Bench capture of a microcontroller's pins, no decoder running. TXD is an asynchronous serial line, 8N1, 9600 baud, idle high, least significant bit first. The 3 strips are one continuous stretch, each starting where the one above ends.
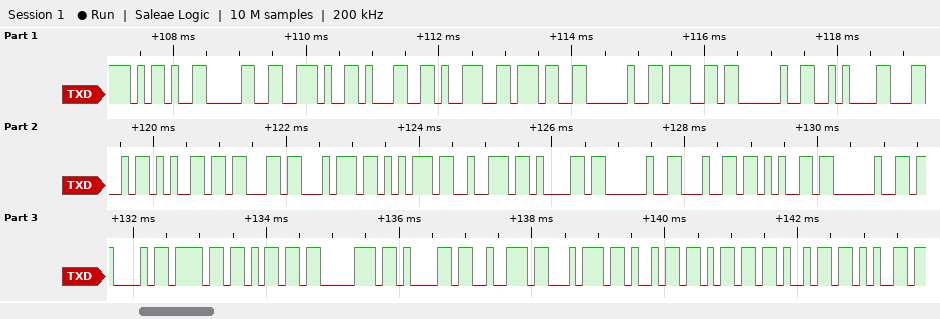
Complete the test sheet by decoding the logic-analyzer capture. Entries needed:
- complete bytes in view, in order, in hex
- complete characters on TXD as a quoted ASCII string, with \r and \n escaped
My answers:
0x2D 0x30 0x2E 0x31 0x39 0x37 0x20 0x67 0x20 0x0A 0x4C 0x65 0x63 0x74 0x75 0x72 0x61 0x20 0x64 0x65 0x20 0x43 0x6F 0x6D 0x70 0x61 0x72 0x74 0x69 0x6D 0x69 0x65
"-0.197 g \nLectura de Compartimie"
